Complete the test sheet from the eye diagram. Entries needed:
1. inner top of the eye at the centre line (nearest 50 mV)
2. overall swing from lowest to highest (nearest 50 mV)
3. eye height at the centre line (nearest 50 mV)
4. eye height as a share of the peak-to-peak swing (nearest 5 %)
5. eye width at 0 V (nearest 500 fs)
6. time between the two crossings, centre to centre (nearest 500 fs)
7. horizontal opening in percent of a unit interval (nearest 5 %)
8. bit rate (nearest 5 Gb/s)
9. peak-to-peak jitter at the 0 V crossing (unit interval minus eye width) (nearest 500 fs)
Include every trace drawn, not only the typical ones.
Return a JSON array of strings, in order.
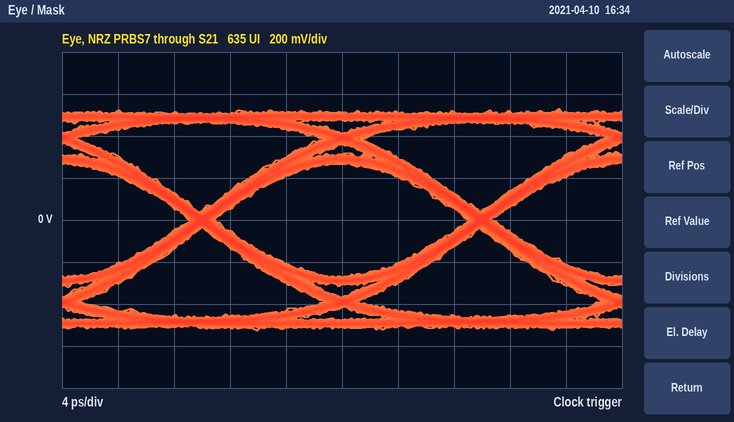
["250 mV", "1.05 V", "550 mV", "50 %", "18.0 ps", "20.0 ps", "90 %", "50 Gb/s", "2.0 ps"]
